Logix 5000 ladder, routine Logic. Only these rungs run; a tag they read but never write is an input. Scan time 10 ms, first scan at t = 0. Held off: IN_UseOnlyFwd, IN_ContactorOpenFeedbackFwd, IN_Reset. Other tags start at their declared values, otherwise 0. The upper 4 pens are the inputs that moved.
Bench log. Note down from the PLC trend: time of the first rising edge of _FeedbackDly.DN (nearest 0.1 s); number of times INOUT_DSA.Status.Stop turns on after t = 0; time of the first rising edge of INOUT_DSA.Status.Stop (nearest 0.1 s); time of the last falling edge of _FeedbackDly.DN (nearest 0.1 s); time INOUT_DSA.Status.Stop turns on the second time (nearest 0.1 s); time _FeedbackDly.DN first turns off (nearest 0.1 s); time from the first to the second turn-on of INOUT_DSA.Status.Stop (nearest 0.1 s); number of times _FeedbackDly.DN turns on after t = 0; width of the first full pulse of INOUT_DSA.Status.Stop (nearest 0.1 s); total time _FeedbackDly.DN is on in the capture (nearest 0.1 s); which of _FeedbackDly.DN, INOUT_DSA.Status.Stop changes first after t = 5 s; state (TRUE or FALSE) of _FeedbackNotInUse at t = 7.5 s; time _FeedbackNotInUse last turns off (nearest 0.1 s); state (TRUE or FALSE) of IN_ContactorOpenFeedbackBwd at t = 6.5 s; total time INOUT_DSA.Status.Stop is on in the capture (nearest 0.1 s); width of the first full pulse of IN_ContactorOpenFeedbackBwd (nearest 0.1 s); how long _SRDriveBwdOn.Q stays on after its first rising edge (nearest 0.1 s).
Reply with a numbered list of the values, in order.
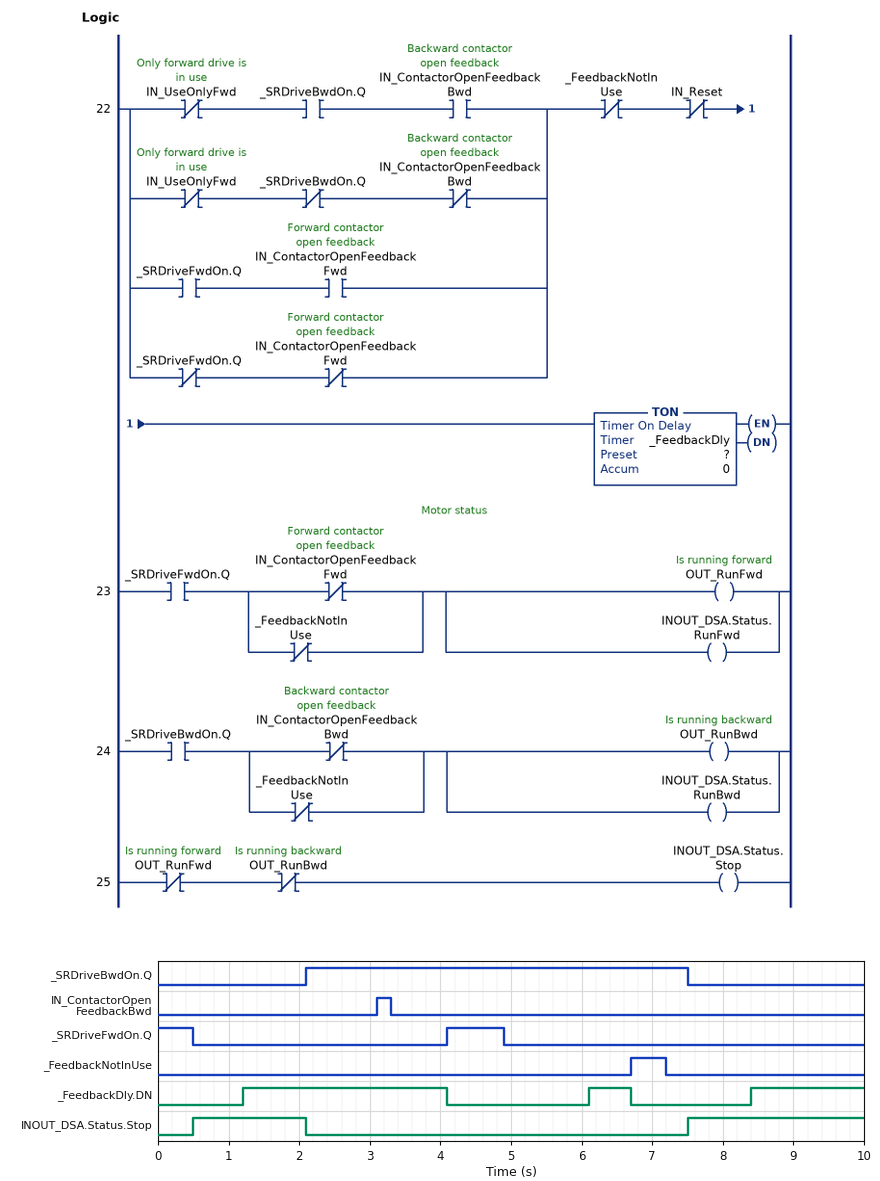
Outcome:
1. 1.2 s
2. 2
3. 0.5 s
4. 6.7 s
5. 7.5 s
6. 4.1 s
7. 7.0 s
8. 3
9. 1.6 s
10. 5.1 s
11. _FeedbackDly.DN
12. FALSE
13. 7.2 s
14. FALSE
15. 4.1 s
16. 0.2 s
17. 5.4 s
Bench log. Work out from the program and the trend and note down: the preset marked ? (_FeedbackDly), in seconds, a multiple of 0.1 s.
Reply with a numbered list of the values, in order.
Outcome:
1. 1.2 s
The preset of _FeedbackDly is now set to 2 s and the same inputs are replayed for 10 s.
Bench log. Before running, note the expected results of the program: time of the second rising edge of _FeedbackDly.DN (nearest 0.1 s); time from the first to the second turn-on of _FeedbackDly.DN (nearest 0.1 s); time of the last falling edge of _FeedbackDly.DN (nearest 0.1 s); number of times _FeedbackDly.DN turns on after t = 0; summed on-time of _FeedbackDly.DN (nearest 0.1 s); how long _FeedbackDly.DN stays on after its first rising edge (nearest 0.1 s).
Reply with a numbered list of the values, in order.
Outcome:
1. 9.2 s
2. 7.2 s
3. 4.1 s
4. 2
5. 2.9 s
6. 2.1 s
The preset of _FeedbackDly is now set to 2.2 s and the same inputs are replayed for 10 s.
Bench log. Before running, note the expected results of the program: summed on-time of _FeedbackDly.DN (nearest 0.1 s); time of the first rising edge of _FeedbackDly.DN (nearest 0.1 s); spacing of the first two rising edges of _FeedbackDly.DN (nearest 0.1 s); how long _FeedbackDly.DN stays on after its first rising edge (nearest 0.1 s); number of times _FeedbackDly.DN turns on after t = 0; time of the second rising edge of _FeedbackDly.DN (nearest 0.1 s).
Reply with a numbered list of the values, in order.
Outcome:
1. 2.5 s
2. 2.2 s
3. 7.2 s
4. 1.9 s
5. 2
6. 9.4 s
